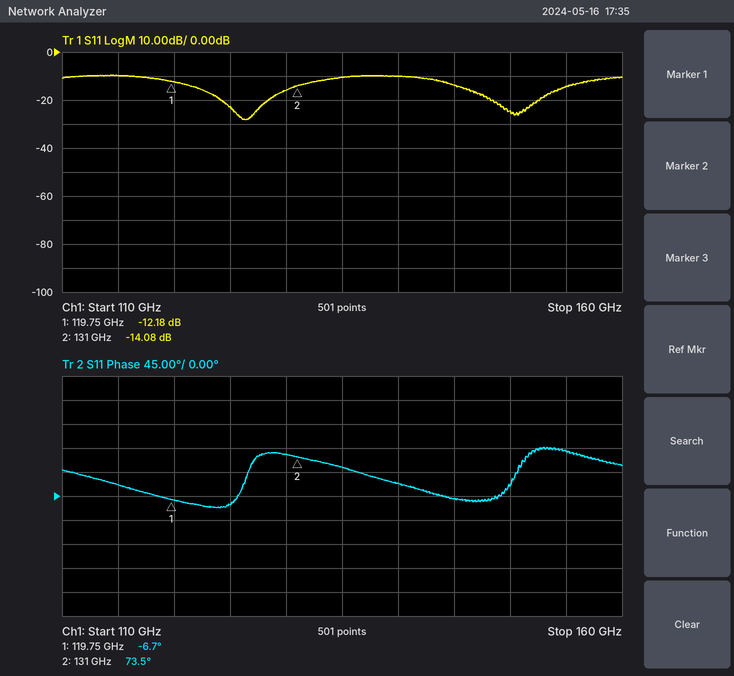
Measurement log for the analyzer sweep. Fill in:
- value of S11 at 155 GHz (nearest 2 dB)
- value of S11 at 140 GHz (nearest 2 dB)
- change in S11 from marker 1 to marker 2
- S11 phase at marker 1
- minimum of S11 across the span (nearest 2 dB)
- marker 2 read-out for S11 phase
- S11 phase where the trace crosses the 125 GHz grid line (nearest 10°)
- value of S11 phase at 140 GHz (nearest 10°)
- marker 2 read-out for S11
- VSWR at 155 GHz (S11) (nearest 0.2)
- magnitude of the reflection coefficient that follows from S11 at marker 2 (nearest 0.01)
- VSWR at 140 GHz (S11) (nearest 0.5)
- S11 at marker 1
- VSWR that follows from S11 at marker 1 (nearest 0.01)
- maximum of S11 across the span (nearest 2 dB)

-14 dB
-10 dB
-1.90 dB
-6.7°
-28 dB
73.5°
-20°
20°
-14.08 dB
1.4
0.20
2.0
-12.18 dB
1.65
-10 dB
